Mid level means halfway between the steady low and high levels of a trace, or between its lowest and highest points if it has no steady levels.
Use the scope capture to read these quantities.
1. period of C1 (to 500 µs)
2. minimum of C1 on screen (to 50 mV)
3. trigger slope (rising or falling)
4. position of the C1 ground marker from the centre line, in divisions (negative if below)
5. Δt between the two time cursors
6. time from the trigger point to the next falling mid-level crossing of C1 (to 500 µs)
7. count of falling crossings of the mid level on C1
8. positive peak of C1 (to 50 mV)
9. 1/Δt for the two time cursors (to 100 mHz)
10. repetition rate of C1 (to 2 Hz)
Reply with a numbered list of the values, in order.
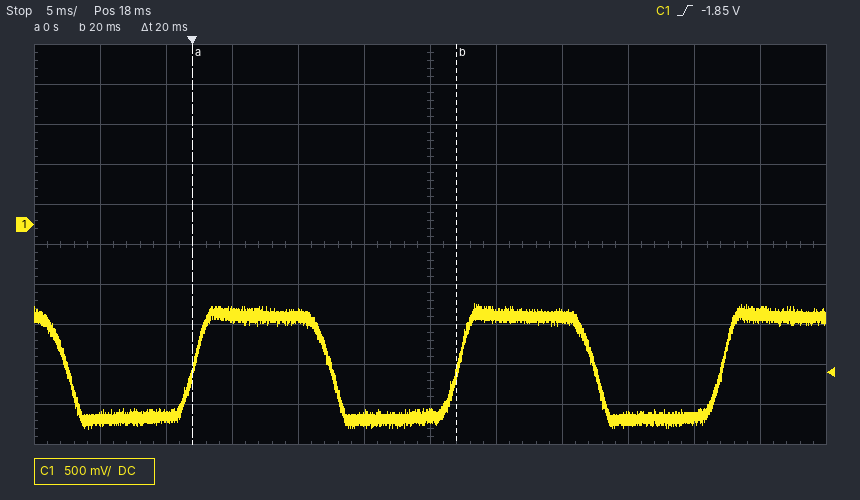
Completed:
1. 20.0 ms
2. -2.55 V
3. rising
4. +0.5 div
5. 20 ms
6. 10.5 ms
7. 3
8. -1.00 V
9. 50.0 Hz
10. 50 Hz
